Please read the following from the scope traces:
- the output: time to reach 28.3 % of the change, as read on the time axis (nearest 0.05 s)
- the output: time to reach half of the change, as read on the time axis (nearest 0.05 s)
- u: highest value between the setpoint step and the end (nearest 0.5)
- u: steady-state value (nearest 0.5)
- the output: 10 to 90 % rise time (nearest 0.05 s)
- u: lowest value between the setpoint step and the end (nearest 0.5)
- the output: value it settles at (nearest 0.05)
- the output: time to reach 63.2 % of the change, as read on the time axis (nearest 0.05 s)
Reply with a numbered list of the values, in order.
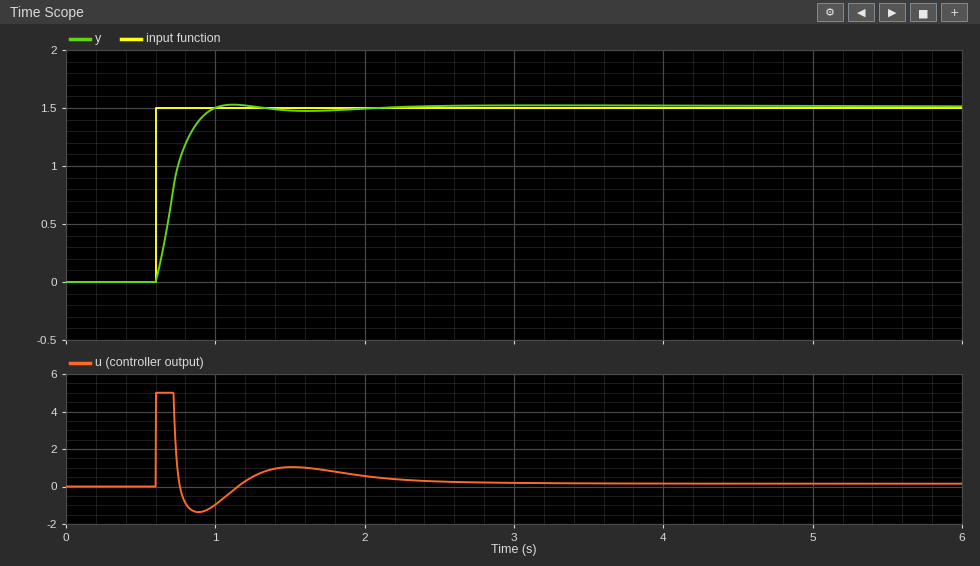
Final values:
1. 0.65 s
2. 0.70 s
3. 5.0
4. 0.0
5. 0.25 s
6. -1.5
7. 1.50
8. 0.75 s
